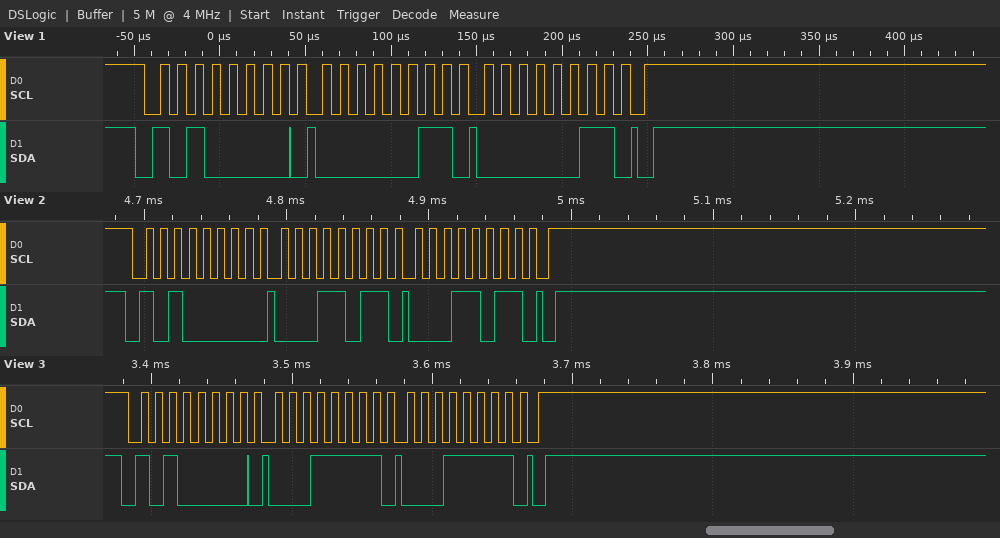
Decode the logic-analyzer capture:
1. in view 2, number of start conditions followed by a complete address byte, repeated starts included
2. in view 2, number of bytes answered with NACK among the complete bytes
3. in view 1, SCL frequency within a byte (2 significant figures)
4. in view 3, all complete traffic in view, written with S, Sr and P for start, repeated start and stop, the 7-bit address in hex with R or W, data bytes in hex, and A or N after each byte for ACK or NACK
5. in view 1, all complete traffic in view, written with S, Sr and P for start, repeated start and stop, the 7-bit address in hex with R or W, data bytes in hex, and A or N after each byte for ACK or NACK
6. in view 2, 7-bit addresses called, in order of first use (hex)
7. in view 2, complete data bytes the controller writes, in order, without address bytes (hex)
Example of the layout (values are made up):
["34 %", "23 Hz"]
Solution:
["1", "0", "100 kHz", "S 50W A 1F A 1F A P", "S 50W A 03 A 03 A P", "0x50", "1B 1B"]
